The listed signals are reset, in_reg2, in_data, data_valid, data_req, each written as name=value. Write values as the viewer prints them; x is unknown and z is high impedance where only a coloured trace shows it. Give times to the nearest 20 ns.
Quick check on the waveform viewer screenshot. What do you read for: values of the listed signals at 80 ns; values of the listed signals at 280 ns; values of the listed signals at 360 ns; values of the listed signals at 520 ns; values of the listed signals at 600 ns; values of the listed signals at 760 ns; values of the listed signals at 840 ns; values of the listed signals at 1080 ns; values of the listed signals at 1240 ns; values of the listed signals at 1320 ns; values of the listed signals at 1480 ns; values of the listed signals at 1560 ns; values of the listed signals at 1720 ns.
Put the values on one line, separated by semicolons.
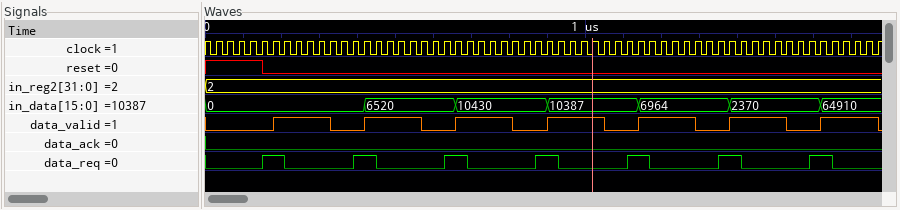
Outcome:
reset=1, in_reg2=2, in_data=0, data_valid=0, data_req=0; reset=0, in_reg2=2, in_data=0, data_valid=1, data_req=0; reset=0, in_reg2=2, in_data=0, data_valid=0, data_req=0; reset=0, in_reg2=2, in_data=6520, data_valid=1, data_req=0; reset=0, in_reg2=2, in_data=6520, data_valid=0, data_req=0; reset=0, in_reg2=2, in_data=10430, data_valid=1, data_req=0; reset=0, in_reg2=2, in_data=10430, data_valid=0, data_req=0; reset=0, in_reg2=2, in_data=10387, data_valid=0, data_req=0; reset=0, in_reg2=2, in_data=6964, data_valid=1, data_req=0; reset=0, in_reg2=2, in_data=6964, data_valid=0, data_req=0; reset=0, in_reg2=2, in_data=2370, data_valid=1, data_req=0; reset=0, in_reg2=2, in_data=2370, data_valid=0, data_req=0; reset=0, in_reg2=2, in_data=64910, data_valid=1, data_req=0
